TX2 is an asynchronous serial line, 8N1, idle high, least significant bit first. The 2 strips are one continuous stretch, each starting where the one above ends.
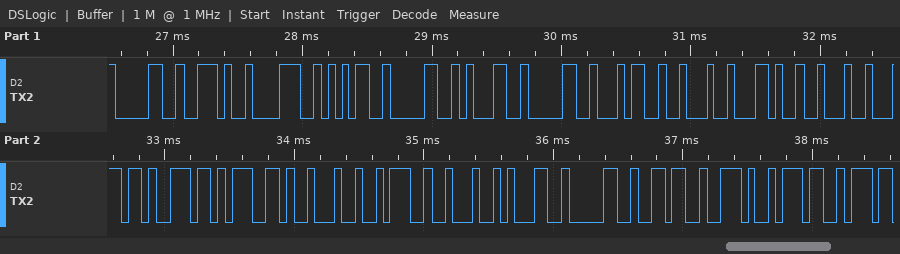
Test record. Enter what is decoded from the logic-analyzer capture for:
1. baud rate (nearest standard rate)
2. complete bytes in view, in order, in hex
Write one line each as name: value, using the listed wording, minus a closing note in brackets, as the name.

baud rate: 19200 baud
complete bytes in view, in order, in hex: 30 2E 38 35 30 31 30 34 22 2C 22 6C 6E 67 22 3A 22 31 30 36 2E 37
